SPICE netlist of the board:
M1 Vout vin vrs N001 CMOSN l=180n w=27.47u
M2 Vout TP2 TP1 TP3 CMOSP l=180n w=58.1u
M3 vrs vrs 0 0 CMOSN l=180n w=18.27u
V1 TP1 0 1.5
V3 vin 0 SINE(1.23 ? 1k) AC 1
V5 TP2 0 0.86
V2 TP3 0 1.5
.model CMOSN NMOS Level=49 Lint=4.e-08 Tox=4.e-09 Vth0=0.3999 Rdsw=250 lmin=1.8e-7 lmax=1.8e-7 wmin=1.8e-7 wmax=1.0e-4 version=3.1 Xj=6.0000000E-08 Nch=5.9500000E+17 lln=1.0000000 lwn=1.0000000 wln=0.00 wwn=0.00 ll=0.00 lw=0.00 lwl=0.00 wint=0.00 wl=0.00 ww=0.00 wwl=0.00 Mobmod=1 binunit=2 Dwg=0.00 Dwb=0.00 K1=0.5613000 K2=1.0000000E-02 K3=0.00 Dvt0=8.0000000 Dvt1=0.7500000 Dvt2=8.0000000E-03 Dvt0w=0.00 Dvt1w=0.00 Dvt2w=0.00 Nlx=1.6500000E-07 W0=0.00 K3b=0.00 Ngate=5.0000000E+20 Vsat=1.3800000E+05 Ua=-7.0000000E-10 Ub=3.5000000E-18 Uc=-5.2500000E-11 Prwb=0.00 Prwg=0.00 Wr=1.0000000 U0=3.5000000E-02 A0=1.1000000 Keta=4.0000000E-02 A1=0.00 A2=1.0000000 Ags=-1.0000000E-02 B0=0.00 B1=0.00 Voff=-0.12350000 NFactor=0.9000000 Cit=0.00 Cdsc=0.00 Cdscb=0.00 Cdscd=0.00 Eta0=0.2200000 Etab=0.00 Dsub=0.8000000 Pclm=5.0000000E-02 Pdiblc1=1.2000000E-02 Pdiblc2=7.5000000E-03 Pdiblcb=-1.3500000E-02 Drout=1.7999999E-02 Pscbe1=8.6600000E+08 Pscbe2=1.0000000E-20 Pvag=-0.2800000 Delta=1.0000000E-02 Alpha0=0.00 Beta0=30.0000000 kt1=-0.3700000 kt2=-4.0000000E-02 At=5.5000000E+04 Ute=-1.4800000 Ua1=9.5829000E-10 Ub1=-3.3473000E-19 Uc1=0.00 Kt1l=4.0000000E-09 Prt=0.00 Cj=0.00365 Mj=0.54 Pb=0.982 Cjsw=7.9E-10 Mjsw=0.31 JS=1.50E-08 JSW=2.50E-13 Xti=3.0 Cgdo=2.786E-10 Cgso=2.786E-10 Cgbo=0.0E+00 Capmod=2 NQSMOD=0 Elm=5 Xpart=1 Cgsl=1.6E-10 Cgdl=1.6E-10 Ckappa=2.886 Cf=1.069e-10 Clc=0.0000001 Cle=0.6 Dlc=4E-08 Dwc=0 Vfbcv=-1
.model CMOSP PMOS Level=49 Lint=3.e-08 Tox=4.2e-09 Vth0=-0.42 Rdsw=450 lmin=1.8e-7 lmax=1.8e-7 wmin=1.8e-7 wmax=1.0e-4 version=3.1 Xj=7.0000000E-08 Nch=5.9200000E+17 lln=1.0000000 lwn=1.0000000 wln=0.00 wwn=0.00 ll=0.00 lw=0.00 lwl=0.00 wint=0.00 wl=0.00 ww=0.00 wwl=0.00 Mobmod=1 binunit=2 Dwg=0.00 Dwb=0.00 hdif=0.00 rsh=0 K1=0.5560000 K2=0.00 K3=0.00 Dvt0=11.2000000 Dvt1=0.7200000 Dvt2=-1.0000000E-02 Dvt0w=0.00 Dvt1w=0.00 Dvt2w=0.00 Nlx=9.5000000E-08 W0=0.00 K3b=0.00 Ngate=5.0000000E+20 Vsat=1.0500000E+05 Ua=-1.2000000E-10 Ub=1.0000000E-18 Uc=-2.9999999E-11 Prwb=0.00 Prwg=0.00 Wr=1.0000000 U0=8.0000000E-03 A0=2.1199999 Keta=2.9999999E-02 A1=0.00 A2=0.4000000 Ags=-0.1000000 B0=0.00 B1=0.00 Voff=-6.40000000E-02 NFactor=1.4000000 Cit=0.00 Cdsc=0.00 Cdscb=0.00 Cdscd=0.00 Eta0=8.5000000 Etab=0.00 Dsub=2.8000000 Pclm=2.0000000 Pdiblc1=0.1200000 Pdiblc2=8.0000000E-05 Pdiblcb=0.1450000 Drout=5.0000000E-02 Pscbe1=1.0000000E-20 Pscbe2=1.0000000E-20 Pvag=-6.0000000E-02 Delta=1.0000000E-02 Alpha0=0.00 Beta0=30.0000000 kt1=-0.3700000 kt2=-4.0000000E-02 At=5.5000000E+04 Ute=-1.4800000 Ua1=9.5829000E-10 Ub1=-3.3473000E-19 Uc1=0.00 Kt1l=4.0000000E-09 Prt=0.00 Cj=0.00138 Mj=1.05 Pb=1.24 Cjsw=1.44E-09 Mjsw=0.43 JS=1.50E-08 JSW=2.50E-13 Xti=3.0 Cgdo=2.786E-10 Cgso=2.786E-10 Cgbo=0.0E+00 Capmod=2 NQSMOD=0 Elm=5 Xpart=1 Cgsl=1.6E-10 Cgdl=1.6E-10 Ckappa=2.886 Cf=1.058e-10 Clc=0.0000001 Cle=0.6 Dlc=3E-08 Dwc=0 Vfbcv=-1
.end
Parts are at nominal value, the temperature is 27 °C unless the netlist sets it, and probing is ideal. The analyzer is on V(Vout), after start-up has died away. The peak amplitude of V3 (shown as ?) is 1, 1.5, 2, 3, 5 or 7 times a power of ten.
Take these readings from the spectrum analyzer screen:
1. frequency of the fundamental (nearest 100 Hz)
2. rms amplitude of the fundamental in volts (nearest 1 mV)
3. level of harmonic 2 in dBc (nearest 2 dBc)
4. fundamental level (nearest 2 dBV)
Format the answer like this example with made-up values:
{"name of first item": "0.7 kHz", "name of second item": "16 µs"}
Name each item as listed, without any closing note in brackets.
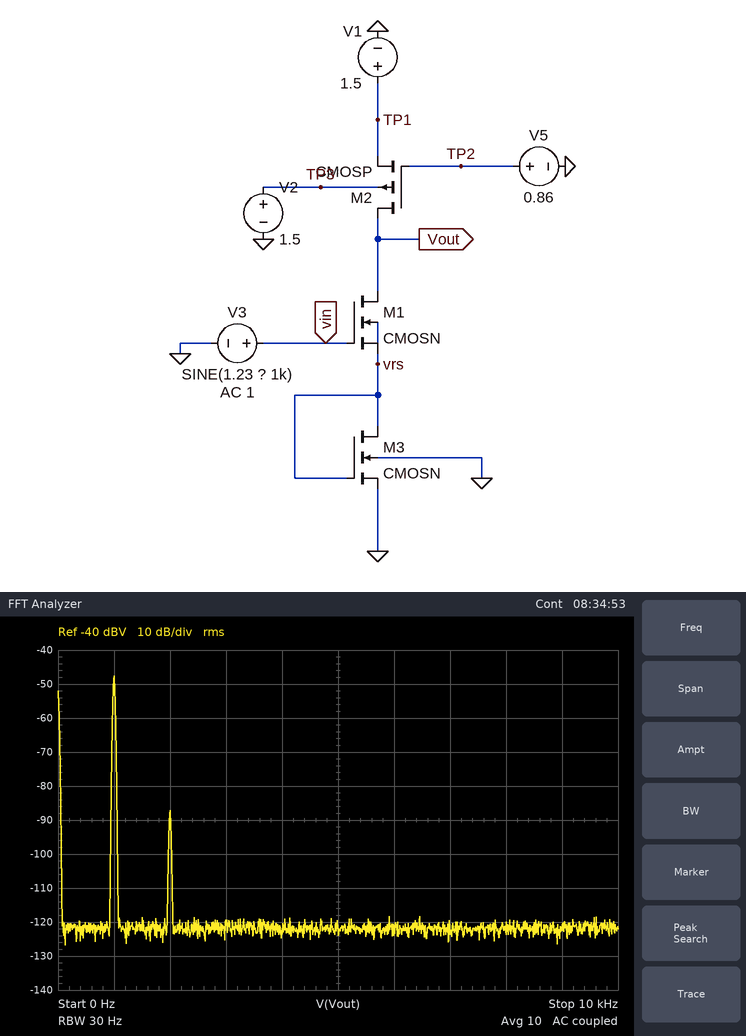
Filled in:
{"frequency of the fundamental": "1.0 kHz", "rms amplitude of the fundamental in volts": "4 mV", "level of harmonic 2 in dBc": "-40 dBc", "fundamental level": "-48 dBV"}
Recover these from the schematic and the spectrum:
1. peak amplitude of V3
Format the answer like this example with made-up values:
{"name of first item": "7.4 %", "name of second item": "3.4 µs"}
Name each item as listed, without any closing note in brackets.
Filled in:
{"peak amplitude of V3": "5 mV"}
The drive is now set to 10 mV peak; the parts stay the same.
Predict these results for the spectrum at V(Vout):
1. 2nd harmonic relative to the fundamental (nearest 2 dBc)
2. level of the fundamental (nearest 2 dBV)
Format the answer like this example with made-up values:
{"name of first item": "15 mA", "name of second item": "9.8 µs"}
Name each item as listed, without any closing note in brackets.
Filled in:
{"2nd harmonic relative to the fundamental": "-34 dBc", "level of the fundamental": "-42 dBV"}
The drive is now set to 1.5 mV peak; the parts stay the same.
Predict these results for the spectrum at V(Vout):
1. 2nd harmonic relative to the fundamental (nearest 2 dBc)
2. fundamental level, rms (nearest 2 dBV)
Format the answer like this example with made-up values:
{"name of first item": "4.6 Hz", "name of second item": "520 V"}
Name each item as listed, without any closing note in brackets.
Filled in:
{"2nd harmonic relative to the fundamental": "-50 dBc", "fundamental level, rms": "-58 dBV"}
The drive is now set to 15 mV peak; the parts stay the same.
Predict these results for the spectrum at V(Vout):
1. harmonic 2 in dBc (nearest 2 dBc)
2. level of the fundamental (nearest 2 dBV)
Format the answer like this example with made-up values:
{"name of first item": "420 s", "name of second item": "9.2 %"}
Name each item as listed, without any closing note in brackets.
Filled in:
{"harmonic 2 in dBc": "-30 dBc", "level of the fundamental": "-38 dBV"}
